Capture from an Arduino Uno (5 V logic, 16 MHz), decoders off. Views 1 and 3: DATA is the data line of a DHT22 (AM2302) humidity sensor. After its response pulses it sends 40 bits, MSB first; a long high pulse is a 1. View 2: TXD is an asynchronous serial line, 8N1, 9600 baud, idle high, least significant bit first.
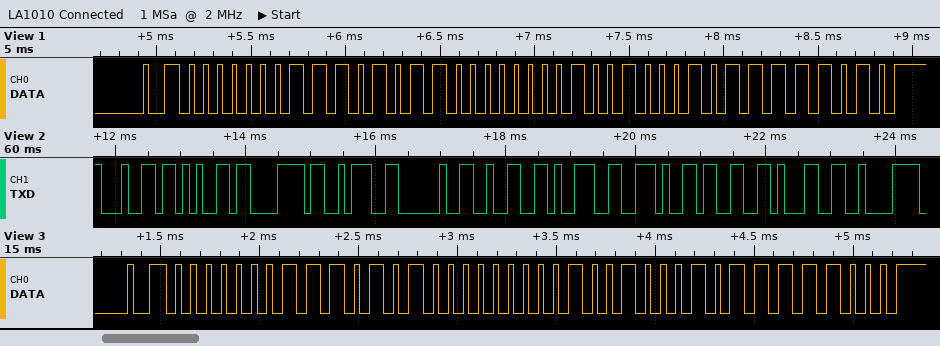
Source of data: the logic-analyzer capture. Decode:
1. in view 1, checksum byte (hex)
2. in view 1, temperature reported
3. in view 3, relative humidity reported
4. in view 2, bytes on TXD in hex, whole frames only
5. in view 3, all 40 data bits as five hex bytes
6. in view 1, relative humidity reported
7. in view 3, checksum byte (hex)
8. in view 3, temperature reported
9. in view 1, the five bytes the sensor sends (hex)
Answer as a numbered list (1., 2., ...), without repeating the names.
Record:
1. 0xFA
2. 29.0 °C
3. 46.8 %
4. 64 65 78 3A 20 32 39 2E 33 31 C2
5. 01 D4 01 22 F8
6. 47.0 %
7. 0xF8
8. 29.0 °C
9. 01 D6 01 22 FA
